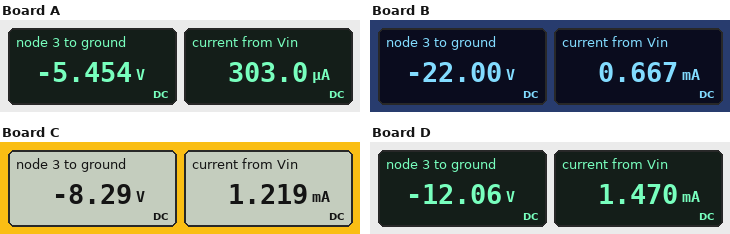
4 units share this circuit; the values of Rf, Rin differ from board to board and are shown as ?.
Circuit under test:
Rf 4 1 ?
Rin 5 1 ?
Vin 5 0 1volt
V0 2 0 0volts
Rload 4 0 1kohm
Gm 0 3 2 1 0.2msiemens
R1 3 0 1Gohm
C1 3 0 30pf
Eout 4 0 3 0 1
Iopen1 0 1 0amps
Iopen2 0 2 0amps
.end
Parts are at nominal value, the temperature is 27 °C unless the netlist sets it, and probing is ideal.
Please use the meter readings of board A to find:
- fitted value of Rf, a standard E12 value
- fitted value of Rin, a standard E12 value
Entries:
18 kΩ
3.3 kΩ
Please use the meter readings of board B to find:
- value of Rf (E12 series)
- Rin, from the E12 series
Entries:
33 kΩ
1.5 kΩ
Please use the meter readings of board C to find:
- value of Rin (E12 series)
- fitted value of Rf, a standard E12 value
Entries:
820 Ω
6.8 kΩ
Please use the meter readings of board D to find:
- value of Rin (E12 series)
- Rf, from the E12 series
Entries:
680 Ω
8.2 kΩ
